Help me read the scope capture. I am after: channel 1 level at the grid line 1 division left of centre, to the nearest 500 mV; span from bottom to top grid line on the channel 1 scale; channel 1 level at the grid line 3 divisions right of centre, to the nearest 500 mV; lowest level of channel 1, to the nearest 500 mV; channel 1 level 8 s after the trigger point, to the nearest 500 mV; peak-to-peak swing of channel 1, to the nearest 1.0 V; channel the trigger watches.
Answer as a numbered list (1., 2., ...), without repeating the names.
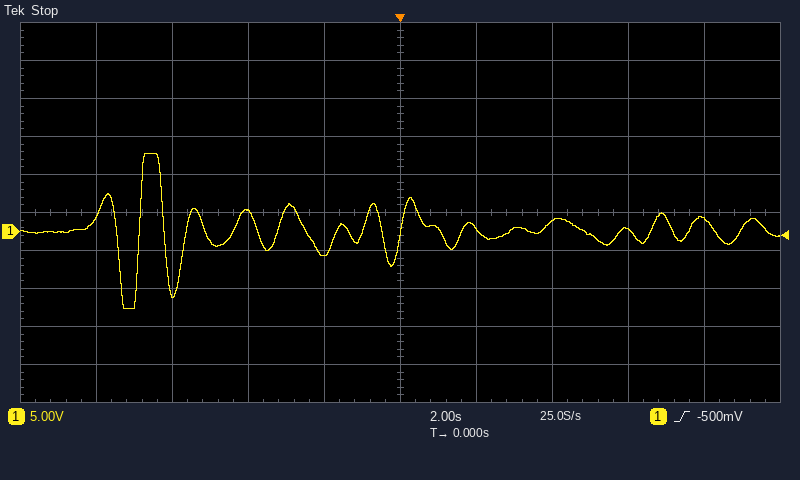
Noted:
1. -3.0 V
2. 50 V
3. 0.0 V
4. -10.0 V
5. 1.5 V
6. 20.0 V
7. channel 1
